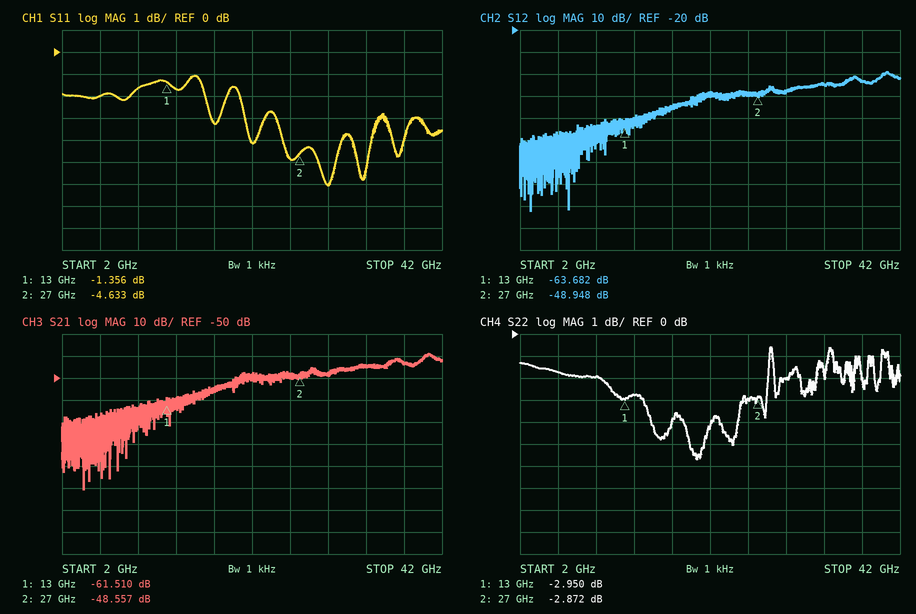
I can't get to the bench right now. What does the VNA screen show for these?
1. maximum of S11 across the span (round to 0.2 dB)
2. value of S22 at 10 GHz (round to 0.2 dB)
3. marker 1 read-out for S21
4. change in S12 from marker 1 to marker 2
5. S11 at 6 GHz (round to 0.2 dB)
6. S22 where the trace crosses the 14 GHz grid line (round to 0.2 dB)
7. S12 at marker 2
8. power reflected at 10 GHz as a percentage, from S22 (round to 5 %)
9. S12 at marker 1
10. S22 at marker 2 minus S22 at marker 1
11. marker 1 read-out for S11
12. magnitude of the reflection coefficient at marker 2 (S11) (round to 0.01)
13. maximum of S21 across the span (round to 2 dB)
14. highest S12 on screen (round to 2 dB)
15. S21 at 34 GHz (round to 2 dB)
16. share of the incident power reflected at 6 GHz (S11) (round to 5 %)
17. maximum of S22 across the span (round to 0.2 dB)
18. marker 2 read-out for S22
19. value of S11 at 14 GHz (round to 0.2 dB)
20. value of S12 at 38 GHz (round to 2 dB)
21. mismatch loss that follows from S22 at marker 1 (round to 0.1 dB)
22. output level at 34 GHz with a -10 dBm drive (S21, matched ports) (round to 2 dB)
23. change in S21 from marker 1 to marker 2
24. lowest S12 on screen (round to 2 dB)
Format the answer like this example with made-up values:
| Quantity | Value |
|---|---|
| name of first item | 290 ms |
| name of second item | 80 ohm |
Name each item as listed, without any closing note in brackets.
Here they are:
| Quantity | Value |
|---|---|
| maximum of S11 across the span | -1.0 dB |
| value of S22 at 10 GHz | -2.0 dB |
| marker 1 read-out for S21 | -61.510 dB |
| change in S12 from marker 1 to marker 2 | 14.734 dB |
| S11 at 6 GHz | -2.0 dB |
| S22 where the trace crosses the 14 GHz grid line | -2.8 dB |
| S12 at marker 2 | -48.948 dB |
| power reflected at 10 GHz as a percentage, from S22 | 65 % |
| S12 at marker 1 | -63.682 dB |
| S22 at marker 2 minus S22 at marker 1 | 0.078 dB |
| marker 1 read-out for S11 | -1.356 dB |
| magnitude of the reflection coefficient at marker 2 (S11) | 0.59 |
| maximum of S21 across the span | -38 dB |
| highest S12 on screen | -38 dB |
| S21 at 34 GHz | -44 dB |
| share of the incident power reflected at 6 GHz (S11) | 65 % |
| maximum of S22 across the span | -0.6 dB |
| marker 2 read-out for S22 | -2.872 dB |
| value of S11 at 14 GHz | -1.6 dB |
| value of S12 at 38 GHz | -44 dB |
| mismatch loss that follows from S22 at marker 1 | 3.1 dB |
| output level at 34 GHz with a -10 dBm drive (S21, matched ports) | -54 dBm |
| change in S21 from marker 1 to marker 2 | 12.953 dB |
| lowest S12 on screen | -102 dB |
